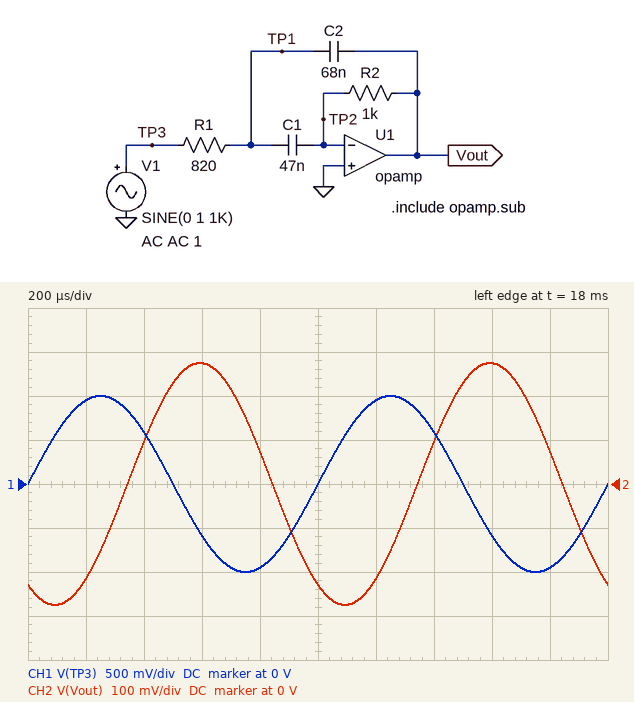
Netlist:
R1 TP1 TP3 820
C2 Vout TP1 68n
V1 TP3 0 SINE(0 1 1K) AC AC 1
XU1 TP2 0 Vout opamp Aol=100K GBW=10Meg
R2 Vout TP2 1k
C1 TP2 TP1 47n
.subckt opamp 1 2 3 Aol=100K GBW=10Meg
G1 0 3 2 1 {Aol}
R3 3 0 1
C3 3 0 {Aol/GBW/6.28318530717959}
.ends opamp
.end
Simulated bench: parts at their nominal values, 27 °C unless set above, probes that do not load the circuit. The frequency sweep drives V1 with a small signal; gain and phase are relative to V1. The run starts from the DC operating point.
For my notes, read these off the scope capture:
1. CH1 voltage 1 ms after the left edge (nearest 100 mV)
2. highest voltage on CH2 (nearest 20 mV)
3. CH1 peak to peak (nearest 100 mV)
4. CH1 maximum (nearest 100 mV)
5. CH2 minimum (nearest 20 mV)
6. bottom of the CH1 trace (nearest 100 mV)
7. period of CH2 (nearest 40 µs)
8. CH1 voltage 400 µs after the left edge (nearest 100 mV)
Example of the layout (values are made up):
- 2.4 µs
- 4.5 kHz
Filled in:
- 0 V
- 280 mV
- 2.0 V
- 1.0 V
- -280 mV
- -1.0 V
- 1.00 ms
- 600 mV
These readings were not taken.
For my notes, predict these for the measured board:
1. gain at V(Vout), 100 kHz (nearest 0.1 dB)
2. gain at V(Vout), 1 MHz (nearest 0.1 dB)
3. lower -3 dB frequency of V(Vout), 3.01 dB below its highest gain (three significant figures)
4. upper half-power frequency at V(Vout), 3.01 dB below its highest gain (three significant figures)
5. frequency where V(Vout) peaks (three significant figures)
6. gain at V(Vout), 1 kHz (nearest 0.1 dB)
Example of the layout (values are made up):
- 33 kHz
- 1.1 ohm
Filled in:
- -30.9 dB
- -50.9 dB
- 1.36 kHz
- 7.09 kHz
- 3.11 kHz
- -11.2 dB
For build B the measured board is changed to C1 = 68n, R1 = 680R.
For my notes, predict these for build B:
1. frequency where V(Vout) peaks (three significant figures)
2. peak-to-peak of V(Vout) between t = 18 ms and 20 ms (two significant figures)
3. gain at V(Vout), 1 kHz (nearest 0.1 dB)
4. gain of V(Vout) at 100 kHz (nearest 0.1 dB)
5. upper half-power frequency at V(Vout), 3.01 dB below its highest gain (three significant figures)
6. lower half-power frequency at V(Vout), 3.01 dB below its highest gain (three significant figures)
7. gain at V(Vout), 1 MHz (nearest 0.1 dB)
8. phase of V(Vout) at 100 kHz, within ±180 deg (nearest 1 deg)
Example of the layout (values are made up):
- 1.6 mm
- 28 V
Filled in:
- 2.84 kHz
- 810 mV
- -7.8 dB
- -29.3 dB
- 6.02 kHz
- 1.34 kHz
- -49.3 dB
- 92 deg
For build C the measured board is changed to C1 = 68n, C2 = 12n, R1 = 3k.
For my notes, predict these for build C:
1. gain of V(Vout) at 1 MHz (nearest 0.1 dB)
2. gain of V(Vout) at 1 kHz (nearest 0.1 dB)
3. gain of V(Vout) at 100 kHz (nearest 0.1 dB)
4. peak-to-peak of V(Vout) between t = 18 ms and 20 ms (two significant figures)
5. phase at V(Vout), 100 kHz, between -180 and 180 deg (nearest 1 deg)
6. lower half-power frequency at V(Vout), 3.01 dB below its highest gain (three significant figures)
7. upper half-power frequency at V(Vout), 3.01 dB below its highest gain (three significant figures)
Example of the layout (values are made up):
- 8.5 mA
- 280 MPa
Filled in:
- -47.1 dB
- -12.3 dB
- -27.2 dB
- 490 mV
- 98 deg
- 637 Hz
- 16.2 kHz
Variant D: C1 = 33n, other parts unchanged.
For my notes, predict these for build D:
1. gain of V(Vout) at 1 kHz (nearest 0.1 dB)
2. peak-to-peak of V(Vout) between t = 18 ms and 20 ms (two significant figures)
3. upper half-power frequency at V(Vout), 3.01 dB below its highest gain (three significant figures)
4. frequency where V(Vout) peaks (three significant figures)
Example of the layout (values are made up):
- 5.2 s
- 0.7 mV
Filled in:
- -14.2 dB
- 390 mV
- 8.74 kHz
- 3.71 kHz
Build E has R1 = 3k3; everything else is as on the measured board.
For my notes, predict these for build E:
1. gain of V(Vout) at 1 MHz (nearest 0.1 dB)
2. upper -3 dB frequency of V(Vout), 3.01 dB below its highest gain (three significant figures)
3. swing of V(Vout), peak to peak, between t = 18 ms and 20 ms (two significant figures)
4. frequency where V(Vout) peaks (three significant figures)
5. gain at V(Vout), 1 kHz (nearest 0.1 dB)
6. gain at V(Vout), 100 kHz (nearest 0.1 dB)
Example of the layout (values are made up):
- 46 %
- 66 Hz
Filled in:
- -63.0 dB
- 6.12 kHz
- 240 mV
- 1.55 kHz
- -18.4 dB
- -43.0 dB
